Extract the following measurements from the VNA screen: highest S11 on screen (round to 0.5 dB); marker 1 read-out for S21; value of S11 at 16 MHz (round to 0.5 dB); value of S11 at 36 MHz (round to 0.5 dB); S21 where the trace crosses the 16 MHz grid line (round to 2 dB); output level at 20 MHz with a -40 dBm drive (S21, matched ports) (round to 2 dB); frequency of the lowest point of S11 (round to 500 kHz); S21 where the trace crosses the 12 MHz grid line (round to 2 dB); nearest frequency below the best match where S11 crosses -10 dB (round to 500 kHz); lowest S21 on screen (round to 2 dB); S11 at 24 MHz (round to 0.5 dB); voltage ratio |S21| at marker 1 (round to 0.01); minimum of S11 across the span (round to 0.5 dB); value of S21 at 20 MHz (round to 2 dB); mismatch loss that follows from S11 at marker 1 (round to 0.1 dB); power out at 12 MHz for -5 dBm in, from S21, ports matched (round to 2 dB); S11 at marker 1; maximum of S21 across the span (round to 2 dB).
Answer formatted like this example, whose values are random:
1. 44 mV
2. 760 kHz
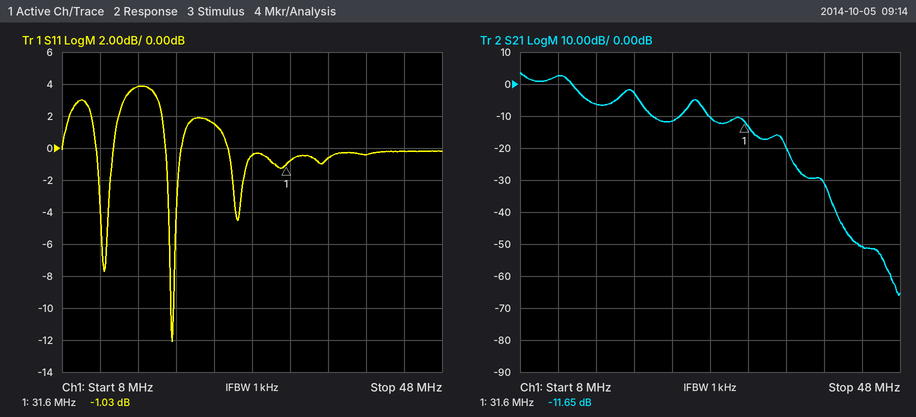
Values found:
1. 4.0 dB
2. -11.65 dB
3. 4.0 dB
4. -0.5 dB
5. -6 dB
6. -42 dBm
7. 19.5 MHz
8. 2 dB
9. 19.5 MHz
10. -66 dB
11. 1.5 dB
12. 0.26
13. -12.0 dB
14. -2 dB
15. 6.8 dB
16. -2 dBm
17. -1.03 dB
18. 4 dB
